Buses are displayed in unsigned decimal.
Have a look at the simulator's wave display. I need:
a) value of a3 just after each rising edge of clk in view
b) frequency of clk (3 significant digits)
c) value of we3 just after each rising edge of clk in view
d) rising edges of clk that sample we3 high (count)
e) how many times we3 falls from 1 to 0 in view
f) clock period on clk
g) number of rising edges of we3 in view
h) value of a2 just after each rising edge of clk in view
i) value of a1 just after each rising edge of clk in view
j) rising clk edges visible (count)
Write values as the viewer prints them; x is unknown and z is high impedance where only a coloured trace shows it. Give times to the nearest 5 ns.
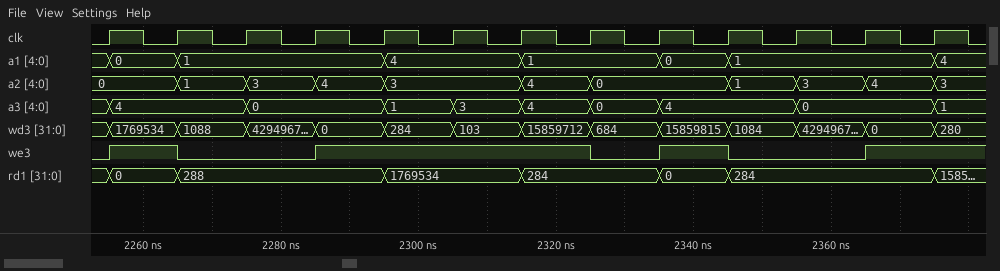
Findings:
4, 4, 0, 0, 1, 3, 4, 0, 4, 4, 0, 0, 1
100 MHz
1 0 0 1 1 1 1 0 1 0 0 1 1
7
3
10 ns
4
0, 1, 3, 4, 3, 3, 4, 0, 0, 1, 3, 4, 3
0, 1, 1, 1, 4, 4, 1, 1, 0, 1, 1, 1, 4
13
